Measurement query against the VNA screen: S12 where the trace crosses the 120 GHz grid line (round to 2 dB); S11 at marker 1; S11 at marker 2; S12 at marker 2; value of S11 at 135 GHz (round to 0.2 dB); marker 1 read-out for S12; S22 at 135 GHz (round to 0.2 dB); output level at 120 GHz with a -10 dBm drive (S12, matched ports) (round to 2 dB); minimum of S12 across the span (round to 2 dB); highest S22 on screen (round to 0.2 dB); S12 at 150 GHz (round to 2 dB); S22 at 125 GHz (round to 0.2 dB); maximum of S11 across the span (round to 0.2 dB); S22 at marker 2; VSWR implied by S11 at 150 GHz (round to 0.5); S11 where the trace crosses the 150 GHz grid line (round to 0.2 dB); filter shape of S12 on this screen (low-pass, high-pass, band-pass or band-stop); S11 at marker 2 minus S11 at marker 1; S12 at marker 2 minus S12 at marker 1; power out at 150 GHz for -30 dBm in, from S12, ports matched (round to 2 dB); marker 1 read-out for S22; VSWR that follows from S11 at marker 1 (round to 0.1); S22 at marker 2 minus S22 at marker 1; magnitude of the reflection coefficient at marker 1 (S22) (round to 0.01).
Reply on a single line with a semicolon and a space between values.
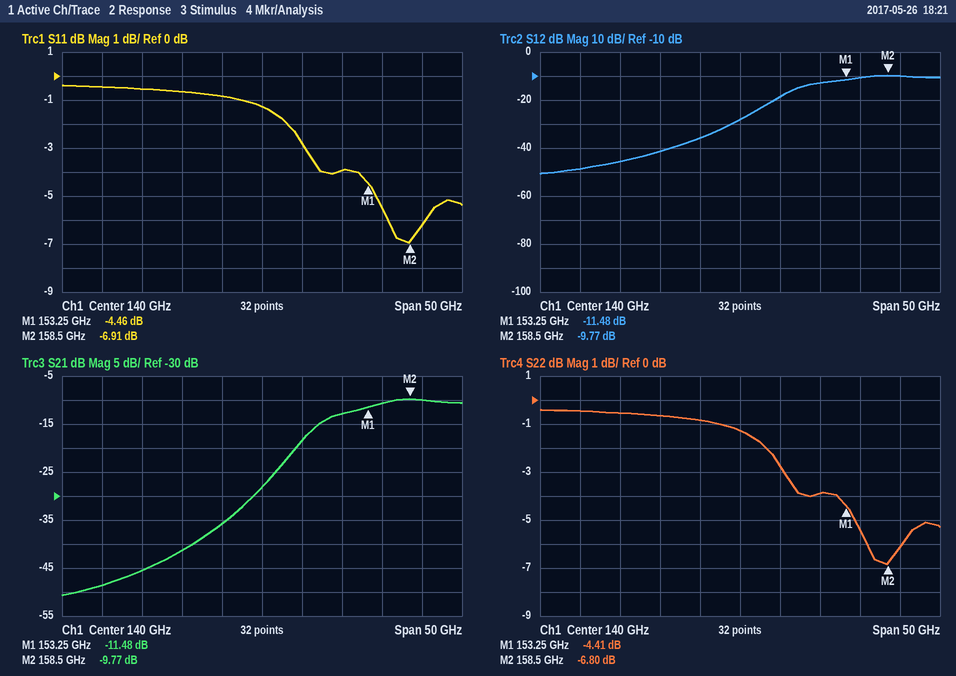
-48 dB; -4.46 dB; -6.91 dB; -9.77 dB; -0.8 dB; -11.48 dB; -0.8 dB; -58 dBm; -50 dB; -0.4 dB; -12 dB; -0.6 dB; -0.4 dB; -6.80 dB; 4.5; -4.0 dB; high-pass; -2.45 dB; 1.71 dB; -42 dBm; -4.41 dB; 4.0; -2.39 dB; 0.60
